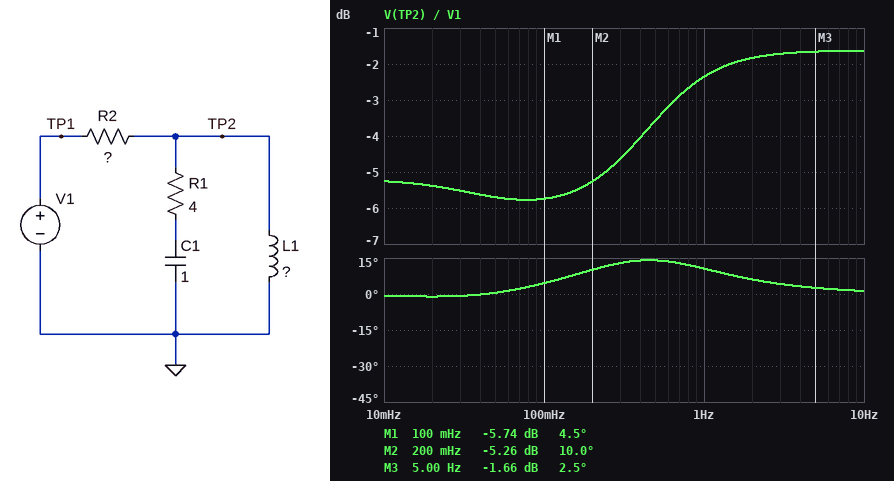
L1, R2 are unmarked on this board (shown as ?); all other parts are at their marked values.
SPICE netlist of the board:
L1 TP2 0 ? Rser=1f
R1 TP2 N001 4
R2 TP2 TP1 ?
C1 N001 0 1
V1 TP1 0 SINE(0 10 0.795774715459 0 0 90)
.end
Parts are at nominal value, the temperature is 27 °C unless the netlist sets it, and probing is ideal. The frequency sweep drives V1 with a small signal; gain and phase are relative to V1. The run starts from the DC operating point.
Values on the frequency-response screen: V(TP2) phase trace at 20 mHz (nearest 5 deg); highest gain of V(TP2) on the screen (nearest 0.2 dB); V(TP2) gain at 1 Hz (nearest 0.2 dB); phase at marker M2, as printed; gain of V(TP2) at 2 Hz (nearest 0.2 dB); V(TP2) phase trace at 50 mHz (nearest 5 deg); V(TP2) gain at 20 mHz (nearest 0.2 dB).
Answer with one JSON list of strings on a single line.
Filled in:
["0 deg", "-1.6 dB", "-2.4 dB", "10.0 deg", "-1.8 dB", "0 deg", "-5.4 dB"]
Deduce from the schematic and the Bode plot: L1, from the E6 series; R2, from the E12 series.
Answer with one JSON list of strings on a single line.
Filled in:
["470 mH", "0.82 Ω"]
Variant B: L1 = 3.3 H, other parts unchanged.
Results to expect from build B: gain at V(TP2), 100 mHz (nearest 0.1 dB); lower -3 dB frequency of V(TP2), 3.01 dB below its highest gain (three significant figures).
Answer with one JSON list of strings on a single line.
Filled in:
["-2.6 dB", "27.6 mHz"]
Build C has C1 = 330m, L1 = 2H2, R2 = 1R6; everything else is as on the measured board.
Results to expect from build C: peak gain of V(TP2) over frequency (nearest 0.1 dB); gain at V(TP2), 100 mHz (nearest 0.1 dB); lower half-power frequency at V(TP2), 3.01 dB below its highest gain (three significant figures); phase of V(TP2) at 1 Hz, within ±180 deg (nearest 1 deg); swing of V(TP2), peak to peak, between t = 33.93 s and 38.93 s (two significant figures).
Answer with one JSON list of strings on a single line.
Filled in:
["-2.9 dB", "-5.1 dB", "75.3 mHz", "3 deg", "14 V"]
